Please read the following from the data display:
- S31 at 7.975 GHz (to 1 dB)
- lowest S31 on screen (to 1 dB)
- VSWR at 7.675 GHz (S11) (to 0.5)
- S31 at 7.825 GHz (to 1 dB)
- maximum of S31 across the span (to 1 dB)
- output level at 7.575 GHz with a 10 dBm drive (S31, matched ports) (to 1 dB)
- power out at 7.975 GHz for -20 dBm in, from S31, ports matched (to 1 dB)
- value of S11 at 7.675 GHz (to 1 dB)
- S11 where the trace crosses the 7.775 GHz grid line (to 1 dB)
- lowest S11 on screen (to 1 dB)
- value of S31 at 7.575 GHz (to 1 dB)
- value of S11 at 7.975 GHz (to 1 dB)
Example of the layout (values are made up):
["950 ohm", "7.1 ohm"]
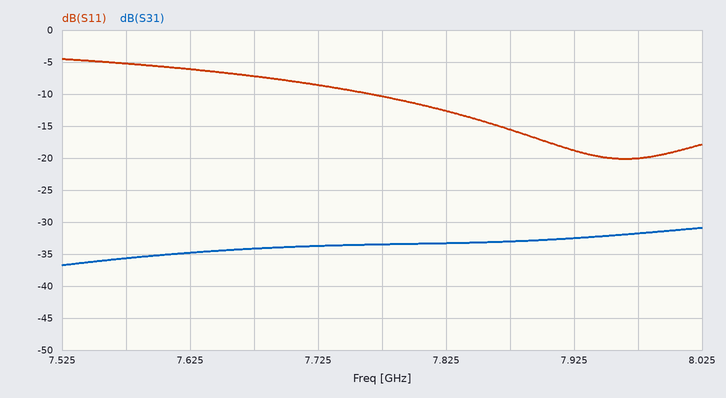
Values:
["-32 dB", "-37 dB", "2.5", "-33 dB", "-31 dB", "-26 dBm", "-52 dBm", "-7 dB", "-10 dB", "-20 dB", "-36 dB", "-20 dB"]
